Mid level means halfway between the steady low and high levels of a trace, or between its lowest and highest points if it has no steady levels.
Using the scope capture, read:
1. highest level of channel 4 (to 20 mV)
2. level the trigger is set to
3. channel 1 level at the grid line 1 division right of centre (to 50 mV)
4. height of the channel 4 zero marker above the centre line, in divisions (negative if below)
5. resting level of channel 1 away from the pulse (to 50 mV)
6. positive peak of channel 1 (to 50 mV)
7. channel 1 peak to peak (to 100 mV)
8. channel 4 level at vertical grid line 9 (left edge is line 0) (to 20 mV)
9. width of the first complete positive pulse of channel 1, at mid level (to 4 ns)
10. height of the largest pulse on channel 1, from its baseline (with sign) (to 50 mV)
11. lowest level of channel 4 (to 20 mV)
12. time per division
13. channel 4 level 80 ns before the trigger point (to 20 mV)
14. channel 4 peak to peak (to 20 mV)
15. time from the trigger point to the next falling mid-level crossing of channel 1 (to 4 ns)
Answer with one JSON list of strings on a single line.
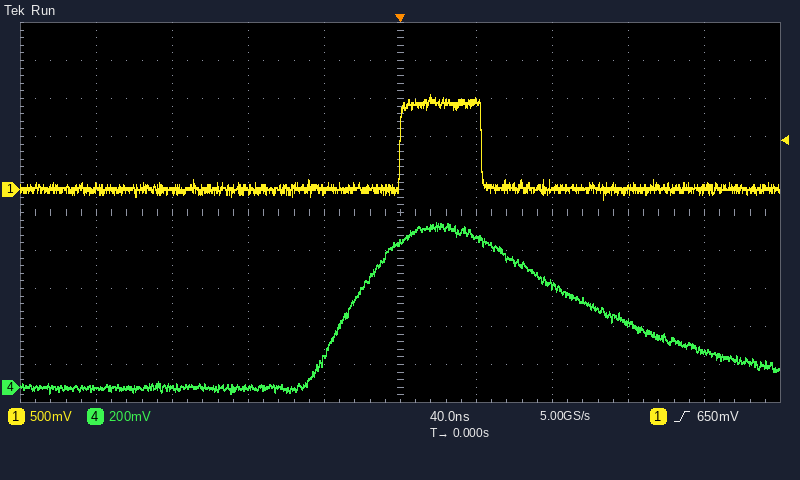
["860 mV", "650 mV", "1.15 V", "-4.6 div", "0 mV", "1.25 V", "1.40 V", "180 mV", "44 ns", "+1.25 V", "-40 mV", "40 ns", "0 mV", "900 mV", "44 ns"]
